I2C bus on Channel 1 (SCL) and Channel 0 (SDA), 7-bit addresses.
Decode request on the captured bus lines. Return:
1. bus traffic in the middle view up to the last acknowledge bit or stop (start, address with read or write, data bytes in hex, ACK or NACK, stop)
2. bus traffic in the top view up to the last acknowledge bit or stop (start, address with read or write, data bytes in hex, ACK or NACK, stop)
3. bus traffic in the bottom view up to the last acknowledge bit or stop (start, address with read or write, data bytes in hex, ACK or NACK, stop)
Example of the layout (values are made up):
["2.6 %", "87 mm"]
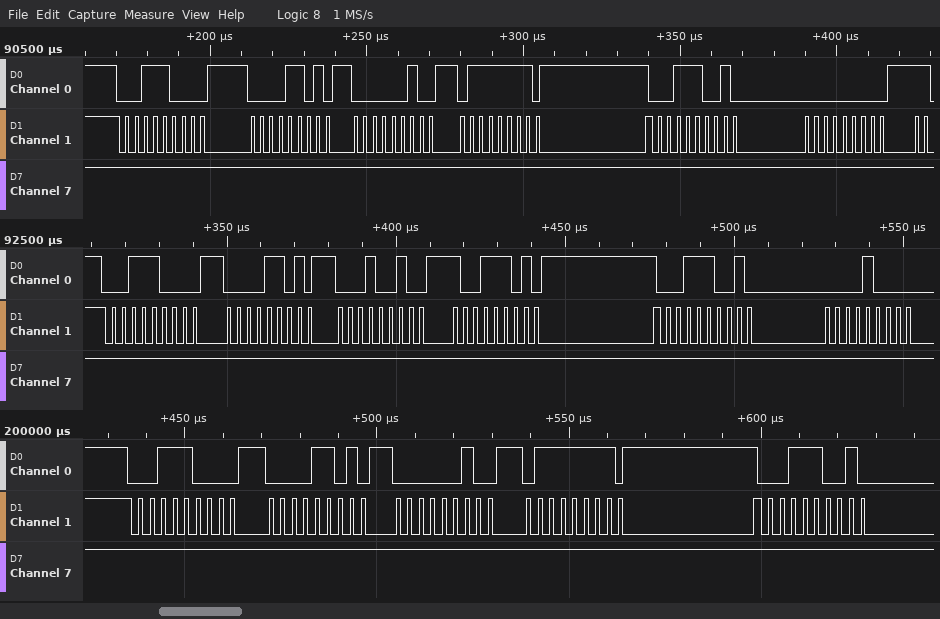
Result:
["start, address 1C write ACK, 0D ACK, 12 ACK, 9D ACK, repeated start, address 1C read ACK, 08 ACK", "start, address 1C write ACK, 0D ACK, 02 ACK, 7F ACK, repeated start, address 1C read ACK, 00 ACK", "start, address 1C write ACK, 0D ACK, 02 ACK, 7F ACK, repeated start, address 1C read ACK"]
